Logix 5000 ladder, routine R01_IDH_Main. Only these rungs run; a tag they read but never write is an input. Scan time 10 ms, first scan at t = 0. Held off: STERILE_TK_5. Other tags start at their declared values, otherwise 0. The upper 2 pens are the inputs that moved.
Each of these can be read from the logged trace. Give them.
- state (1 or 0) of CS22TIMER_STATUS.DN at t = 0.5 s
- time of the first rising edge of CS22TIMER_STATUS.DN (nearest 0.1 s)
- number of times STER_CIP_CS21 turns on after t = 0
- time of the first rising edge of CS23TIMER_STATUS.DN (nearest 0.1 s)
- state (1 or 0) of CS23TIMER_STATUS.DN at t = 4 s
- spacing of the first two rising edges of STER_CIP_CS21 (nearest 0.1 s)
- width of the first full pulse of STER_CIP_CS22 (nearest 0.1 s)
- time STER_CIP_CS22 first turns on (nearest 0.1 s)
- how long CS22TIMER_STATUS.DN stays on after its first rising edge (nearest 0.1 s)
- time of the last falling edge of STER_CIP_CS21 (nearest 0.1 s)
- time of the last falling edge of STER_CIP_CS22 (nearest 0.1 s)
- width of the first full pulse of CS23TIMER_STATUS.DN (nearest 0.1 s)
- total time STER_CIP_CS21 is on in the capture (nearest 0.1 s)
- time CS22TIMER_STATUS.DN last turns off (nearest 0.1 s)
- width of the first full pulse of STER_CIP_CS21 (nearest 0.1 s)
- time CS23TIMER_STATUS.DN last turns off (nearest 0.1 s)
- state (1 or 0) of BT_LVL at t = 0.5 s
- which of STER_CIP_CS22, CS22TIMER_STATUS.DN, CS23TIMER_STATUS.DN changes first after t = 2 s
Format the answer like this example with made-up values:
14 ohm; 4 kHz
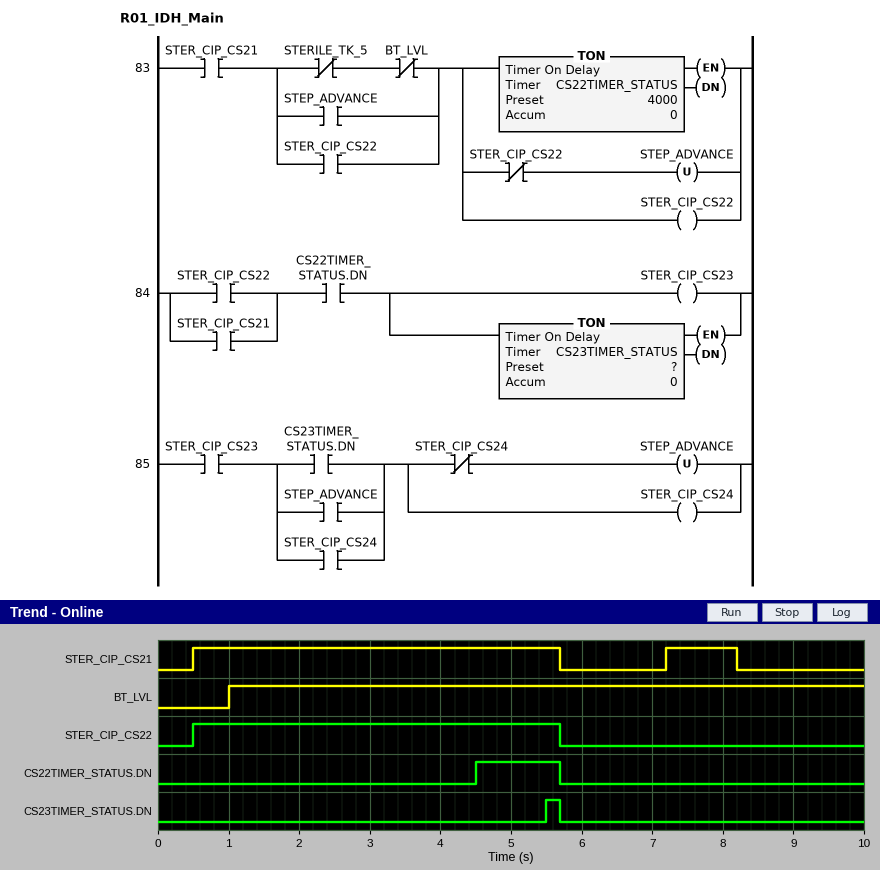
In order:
0; 4.5 s; 2; 5.5 s; 0; 6.7 s; 5.2 s; 0.5 s; 1.2 s; 8.2 s; 5.7 s; 0.2 s; 6.2 s; 5.7 s; 5.2 s; 5.7 s; 0; CS22TIMER_STATUS.DN
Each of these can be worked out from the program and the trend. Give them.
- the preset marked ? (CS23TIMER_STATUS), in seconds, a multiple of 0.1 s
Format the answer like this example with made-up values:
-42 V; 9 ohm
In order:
1.0 s
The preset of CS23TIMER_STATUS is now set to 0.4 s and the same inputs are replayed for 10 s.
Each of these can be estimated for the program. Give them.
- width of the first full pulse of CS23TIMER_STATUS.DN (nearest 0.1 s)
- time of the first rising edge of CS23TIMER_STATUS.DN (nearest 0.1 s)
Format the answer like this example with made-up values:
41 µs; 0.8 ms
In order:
0.8 s; 4.9 s
